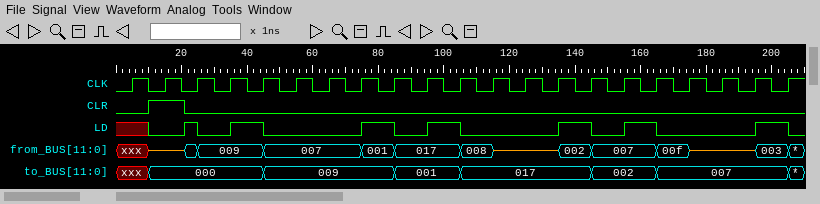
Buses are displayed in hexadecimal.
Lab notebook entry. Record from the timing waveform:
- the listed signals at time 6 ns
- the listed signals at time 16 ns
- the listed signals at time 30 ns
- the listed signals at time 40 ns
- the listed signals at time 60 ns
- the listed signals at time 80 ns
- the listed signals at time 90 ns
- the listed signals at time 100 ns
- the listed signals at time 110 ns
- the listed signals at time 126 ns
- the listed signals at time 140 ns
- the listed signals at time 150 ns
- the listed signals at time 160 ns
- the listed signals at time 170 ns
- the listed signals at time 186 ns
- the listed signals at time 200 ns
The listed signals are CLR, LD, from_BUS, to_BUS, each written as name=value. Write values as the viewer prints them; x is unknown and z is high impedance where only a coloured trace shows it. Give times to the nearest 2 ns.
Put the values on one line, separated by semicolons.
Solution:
CLR=0, LD=x, from_BUS=xxx, to_BUS=xxx; CLR=1, LD=0, from_BUS=z, to_BUS=000; CLR=0, LD=0, from_BUS=009, to_BUS=000; CLR=0, LD=1, from_BUS=009, to_BUS=000; CLR=0, LD=0, from_BUS=007, to_BUS=009; CLR=0, LD=1, from_BUS=001, to_BUS=009; CLR=0, LD=0, from_BUS=017, to_BUS=001; CLR=0, LD=1, from_BUS=017, to_BUS=001; CLR=0, LD=0, from_BUS=008, to_BUS=017; CLR=0, LD=0, from_BUS=z, to_BUS=017; CLR=0, LD=1, from_BUS=002, to_BUS=017; CLR=0, LD=0, from_BUS=007, to_BUS=002; CLR=0, LD=1, from_BUS=007, to_BUS=002; CLR=0, LD=0, from_BUS=00f, to_BUS=007; CLR=0, LD=0, from_BUS=z, to_BUS=007; CLR=0, LD=1, from_BUS=003, to_BUS=007
